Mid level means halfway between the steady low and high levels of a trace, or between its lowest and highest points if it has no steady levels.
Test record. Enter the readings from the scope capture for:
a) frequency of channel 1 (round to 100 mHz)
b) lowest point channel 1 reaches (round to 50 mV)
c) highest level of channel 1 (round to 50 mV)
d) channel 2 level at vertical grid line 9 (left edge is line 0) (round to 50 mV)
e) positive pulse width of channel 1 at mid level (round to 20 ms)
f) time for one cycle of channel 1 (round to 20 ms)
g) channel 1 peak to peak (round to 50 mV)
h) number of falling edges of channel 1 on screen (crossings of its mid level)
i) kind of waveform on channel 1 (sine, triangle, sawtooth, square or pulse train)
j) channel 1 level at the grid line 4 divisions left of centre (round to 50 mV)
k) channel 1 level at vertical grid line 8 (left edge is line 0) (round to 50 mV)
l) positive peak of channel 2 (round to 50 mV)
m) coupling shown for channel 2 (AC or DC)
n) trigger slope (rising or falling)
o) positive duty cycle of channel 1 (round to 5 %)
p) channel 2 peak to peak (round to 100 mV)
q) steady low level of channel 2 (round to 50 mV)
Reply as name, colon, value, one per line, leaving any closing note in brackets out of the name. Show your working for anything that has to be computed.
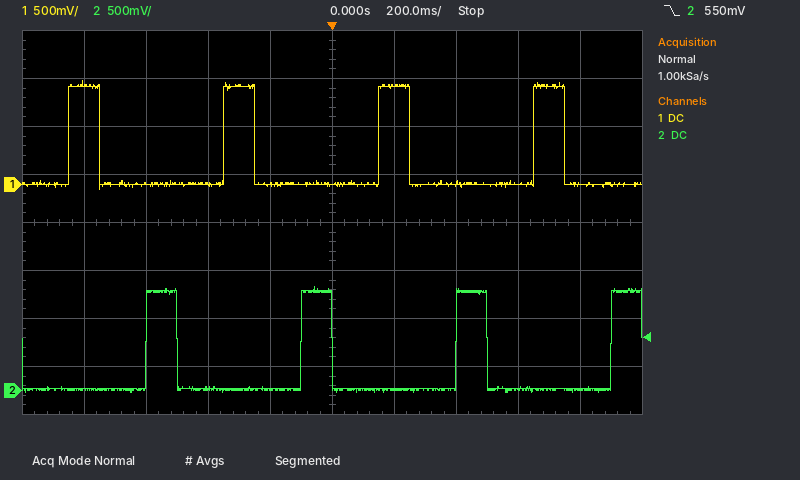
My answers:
frequency of channel 1: 1 / 500 ms ≈ 2.0 Hz
lowest point channel 1 reaches: -50 mV
highest level of channel 1: 1.10 V
channel 2 level at vertical grid line 9 (left edge is line 0): 0 mV
positive pulse width of channel 1 at mid level: 100 ms
time for one cycle of channel 1: 500 ms
channel 1 peak to peak: 1.10 V − (-50 mV) = 1.15 V
number of falling edges of channel 1 on screen: 4
kind of waveform on channel 1: pulse train
channel 1 level at the grid line 4 divisions left of centre: 1.05 V
channel 1 level at vertical grid line 8 (left edge is line 0): 0 mV
positive peak of channel 2: 1.10 V
coupling shown for channel 2: DC
trigger slope: falling
positive duty cycle of channel 1: 100 ms / 500 ms ≈ 20 %
channel 2 peak to peak: 1.10 V
steady low level of channel 2: 0 mV
